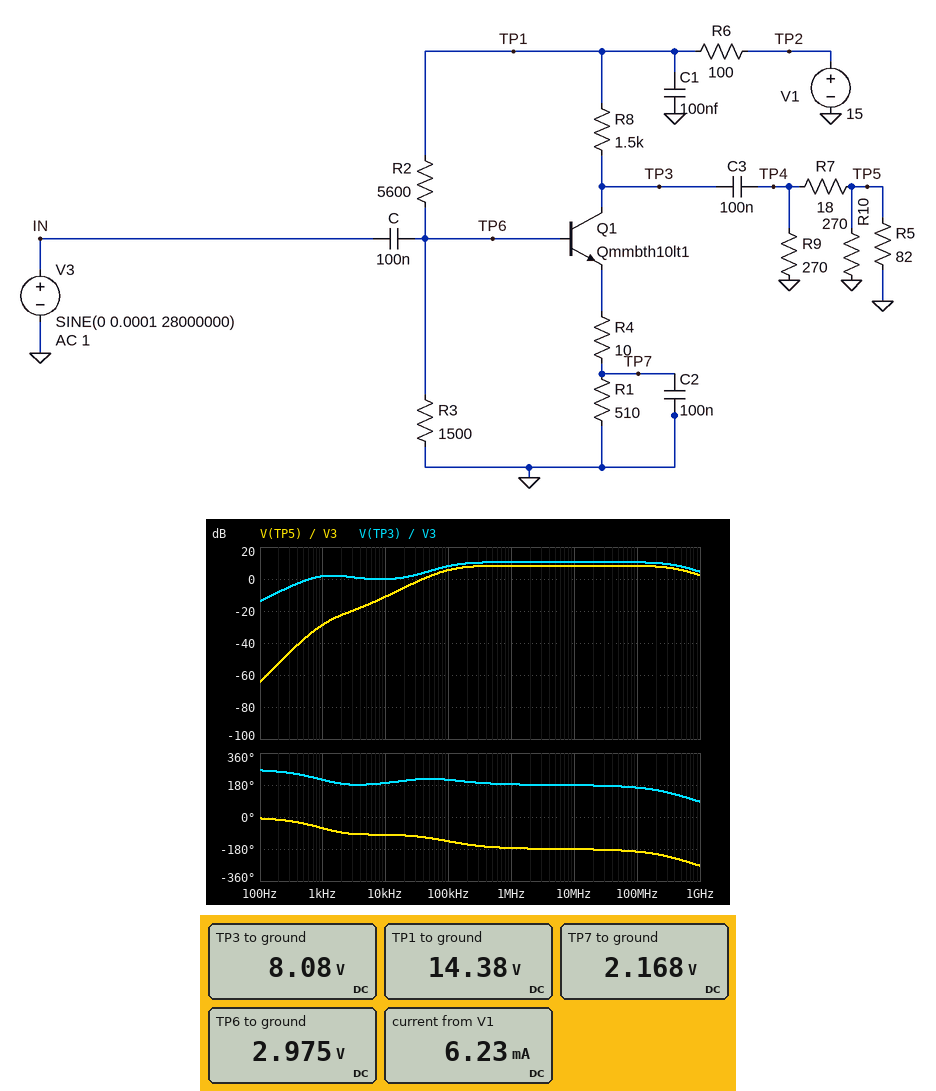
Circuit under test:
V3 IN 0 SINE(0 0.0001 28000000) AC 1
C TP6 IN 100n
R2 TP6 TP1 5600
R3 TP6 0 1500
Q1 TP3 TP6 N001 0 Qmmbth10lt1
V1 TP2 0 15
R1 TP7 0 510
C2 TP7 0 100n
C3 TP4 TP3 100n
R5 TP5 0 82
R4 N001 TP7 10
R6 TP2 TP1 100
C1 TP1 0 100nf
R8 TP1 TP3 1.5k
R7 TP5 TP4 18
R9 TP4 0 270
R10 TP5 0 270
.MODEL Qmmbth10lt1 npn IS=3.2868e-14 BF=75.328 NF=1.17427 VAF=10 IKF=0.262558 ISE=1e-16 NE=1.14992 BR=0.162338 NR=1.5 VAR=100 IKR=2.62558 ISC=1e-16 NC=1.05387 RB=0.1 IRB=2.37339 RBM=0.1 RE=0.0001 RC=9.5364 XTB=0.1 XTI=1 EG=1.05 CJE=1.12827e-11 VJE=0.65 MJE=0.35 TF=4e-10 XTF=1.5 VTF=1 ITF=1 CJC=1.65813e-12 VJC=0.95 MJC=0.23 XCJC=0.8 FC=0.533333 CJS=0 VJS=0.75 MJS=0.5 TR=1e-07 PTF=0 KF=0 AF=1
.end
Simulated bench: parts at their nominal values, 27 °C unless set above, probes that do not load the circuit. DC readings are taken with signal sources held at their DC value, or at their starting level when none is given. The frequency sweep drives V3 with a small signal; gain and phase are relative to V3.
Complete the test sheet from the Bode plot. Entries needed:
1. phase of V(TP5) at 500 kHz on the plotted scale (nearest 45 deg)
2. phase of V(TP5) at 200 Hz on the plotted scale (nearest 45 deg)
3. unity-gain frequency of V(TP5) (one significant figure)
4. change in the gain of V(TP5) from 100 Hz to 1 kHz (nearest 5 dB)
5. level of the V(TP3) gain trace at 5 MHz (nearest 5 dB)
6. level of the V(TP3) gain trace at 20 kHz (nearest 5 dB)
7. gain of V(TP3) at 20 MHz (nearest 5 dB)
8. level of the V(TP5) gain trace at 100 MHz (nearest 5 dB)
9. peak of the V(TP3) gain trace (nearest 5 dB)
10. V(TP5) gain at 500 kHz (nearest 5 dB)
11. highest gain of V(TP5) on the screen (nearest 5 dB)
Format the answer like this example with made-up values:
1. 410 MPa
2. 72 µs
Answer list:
1. -180 deg
2. 0 deg
3. 40 kHz
4. 35 dB
5. 10 dB
6. 0 dB
7. 10 dB
8. 10 dB
9. 10 dB
10. 10 dB
11. 10 dB
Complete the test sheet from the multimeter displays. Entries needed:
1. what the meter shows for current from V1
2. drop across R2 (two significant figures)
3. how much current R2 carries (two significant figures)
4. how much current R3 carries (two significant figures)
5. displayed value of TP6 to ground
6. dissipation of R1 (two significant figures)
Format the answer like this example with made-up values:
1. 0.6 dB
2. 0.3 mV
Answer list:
1. 6.23 mA
2. 11 V
3. 2.0 mA
4. 2.0 mA
5. 2.975 V
6. 9.2 mW
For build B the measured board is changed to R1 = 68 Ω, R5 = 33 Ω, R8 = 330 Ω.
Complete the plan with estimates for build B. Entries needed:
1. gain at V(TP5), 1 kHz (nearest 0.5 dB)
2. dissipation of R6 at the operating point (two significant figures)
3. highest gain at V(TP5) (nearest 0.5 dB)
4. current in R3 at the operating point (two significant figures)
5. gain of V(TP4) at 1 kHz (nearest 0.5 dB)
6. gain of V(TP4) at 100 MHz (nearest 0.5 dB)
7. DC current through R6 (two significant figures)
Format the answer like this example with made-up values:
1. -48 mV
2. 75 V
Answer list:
1. -29.5 dB
2. 47 mW
3. 5.5 dB
4. 1.6 mA
5. -25.5 dB
6. 9.5 dB
7. 22 mA
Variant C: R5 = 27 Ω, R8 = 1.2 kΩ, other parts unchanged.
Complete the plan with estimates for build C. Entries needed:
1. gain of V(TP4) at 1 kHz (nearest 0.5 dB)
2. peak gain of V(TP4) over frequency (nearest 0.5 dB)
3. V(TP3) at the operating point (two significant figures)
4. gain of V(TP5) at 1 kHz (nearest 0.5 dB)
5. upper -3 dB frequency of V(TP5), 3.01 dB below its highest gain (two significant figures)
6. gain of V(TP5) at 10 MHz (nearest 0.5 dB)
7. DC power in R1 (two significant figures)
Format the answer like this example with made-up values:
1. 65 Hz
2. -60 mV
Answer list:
1. -32.0 dB
2. 6.0 dB
3. 9.3 V
4. -36.5 dB
5. 550 MHz
6. 1.5 dB
7. 9.3 mW
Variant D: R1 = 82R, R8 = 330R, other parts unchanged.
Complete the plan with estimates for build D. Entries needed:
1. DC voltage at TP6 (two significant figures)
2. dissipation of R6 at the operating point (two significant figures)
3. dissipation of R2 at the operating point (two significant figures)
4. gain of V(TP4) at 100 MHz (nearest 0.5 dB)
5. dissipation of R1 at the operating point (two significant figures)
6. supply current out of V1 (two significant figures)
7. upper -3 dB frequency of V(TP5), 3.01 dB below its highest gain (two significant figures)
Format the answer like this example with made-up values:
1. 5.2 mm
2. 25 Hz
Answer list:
1. 2.5 V
2. 39 mW
3. 20 mW
4. 12.5 dB
5. 27 mW
6. 20 mA
7. 450 MHz
